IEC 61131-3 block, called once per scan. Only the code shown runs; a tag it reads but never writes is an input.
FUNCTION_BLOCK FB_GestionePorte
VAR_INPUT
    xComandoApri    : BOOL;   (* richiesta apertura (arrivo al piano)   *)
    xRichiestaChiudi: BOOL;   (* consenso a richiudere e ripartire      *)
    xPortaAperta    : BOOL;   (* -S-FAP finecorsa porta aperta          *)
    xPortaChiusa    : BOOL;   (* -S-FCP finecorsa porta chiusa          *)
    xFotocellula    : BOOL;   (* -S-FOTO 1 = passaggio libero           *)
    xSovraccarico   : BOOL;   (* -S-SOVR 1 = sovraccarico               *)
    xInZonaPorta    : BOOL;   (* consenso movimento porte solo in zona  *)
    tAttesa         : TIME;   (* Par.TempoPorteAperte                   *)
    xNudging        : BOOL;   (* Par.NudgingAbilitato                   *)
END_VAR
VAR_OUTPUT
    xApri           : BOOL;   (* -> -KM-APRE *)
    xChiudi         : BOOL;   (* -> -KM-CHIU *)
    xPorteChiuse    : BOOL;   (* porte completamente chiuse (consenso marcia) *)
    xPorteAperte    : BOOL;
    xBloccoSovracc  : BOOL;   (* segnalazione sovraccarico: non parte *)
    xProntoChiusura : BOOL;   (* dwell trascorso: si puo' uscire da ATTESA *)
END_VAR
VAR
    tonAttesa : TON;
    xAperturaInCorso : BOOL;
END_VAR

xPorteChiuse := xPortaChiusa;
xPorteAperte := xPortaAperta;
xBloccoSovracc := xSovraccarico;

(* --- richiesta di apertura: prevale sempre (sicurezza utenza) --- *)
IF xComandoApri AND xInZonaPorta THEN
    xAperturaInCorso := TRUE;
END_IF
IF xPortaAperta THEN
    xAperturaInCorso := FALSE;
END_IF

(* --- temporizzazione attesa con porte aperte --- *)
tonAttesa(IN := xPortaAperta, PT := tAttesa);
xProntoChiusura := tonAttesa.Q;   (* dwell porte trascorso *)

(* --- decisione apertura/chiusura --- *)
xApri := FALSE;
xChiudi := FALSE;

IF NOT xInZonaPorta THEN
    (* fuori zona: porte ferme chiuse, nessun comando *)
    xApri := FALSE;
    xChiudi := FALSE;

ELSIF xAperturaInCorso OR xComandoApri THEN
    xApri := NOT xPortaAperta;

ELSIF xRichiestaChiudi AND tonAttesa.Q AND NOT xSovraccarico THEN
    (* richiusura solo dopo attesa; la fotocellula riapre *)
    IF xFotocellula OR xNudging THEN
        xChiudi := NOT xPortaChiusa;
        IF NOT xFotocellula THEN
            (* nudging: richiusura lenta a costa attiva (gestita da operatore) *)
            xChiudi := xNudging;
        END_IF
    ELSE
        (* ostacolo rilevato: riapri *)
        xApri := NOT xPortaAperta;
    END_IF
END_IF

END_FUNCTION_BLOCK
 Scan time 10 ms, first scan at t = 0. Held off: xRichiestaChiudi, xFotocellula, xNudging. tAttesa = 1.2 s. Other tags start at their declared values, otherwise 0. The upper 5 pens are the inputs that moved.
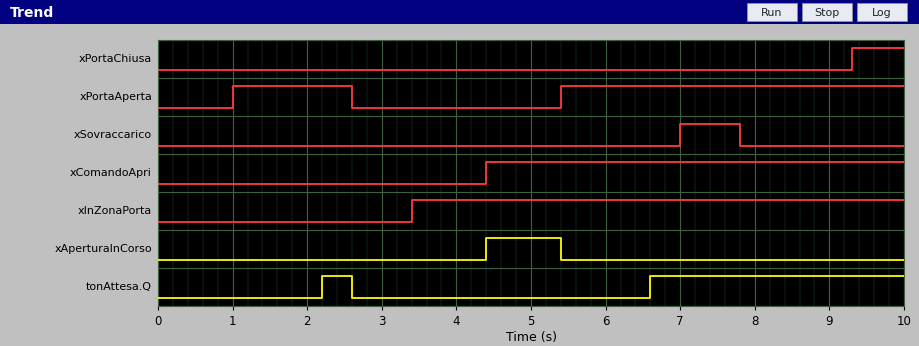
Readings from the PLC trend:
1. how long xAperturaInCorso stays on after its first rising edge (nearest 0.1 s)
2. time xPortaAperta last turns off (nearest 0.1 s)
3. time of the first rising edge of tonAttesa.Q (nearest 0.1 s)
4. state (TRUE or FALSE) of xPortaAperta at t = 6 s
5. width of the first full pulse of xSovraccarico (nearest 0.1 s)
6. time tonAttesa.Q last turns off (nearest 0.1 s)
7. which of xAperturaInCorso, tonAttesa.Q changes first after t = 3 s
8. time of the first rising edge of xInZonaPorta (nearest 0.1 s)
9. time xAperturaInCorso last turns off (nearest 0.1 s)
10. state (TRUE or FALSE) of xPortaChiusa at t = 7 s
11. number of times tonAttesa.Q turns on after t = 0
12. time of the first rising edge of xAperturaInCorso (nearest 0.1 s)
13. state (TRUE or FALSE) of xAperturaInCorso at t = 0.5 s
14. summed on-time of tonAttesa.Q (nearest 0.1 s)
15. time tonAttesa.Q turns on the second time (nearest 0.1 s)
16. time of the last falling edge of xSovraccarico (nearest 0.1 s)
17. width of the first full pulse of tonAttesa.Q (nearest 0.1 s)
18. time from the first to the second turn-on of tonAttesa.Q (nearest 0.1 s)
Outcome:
1.0 s
2.6 s
2.2 s
TRUE
0.8 s
2.6 s
xAperturaInCorso
3.4 s
5.4 s
FALSE
2
4.4 s
FALSE
3.8 s
6.6 s
7.8 s
0.4 s
4.4 s
